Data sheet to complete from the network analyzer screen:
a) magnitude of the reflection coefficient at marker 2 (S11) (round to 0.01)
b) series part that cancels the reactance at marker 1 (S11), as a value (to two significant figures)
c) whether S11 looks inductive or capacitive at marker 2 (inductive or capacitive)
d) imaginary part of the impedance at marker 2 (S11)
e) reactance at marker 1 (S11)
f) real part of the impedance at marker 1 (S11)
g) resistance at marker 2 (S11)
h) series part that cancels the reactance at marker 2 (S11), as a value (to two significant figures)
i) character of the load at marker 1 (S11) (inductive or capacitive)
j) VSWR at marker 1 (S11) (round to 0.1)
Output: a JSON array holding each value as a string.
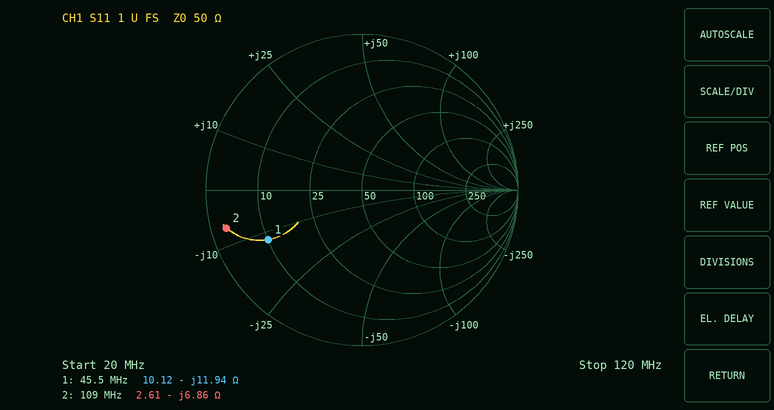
["0.90", "42 nH", "capacitive", "-6.86 Ω", "-11.94 Ω", "10.12 Ω", "2.61 Ω", "10 nH", "capacitive", "5.2"]
